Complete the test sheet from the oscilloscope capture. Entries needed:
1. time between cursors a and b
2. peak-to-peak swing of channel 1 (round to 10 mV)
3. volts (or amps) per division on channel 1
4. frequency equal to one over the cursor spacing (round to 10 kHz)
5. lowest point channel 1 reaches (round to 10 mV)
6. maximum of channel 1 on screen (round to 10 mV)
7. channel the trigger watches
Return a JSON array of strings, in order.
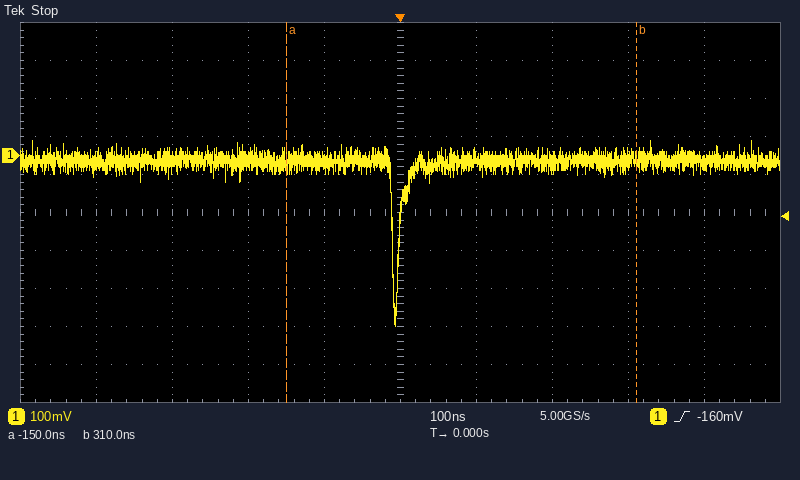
["460 ns", "490 mV", "100 mV", "2.17 MHz", "-450 mV", "40 mV", "channel 1"]
